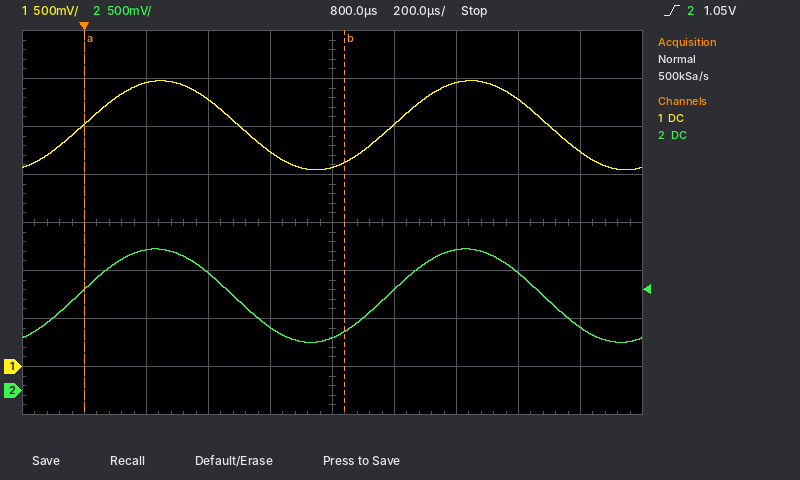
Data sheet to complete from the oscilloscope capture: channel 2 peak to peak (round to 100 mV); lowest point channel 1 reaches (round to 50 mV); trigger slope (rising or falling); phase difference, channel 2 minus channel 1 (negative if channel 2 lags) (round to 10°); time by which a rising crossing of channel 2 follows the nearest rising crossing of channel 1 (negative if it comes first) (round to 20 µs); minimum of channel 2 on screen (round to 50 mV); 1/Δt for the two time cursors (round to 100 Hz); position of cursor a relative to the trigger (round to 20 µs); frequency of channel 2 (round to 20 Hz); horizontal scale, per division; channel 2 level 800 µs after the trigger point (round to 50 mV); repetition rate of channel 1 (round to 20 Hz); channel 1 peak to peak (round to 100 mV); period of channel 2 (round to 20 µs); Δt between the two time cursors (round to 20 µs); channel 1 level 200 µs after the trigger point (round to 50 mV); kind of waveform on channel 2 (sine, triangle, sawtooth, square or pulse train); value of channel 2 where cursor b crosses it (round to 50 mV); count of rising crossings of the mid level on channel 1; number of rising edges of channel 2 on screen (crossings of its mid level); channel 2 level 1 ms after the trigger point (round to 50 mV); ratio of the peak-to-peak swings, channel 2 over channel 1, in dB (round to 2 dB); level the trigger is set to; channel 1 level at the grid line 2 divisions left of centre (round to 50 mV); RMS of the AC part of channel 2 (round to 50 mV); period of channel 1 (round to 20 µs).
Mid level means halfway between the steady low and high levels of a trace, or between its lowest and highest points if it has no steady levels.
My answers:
1.00 V
2.05 V
rising
+10°
-20 µs
500 mV
1.2 kHz
0 µs
1.00 kHz
200 µs
550 mV
1.00 kHz
900 mV
1.00 ms
840 µs
2.95 V
sine
600 mV
2
2
1.05 V
0 dB
1.05 V
2.80 V
350 mV
1.00 ms
